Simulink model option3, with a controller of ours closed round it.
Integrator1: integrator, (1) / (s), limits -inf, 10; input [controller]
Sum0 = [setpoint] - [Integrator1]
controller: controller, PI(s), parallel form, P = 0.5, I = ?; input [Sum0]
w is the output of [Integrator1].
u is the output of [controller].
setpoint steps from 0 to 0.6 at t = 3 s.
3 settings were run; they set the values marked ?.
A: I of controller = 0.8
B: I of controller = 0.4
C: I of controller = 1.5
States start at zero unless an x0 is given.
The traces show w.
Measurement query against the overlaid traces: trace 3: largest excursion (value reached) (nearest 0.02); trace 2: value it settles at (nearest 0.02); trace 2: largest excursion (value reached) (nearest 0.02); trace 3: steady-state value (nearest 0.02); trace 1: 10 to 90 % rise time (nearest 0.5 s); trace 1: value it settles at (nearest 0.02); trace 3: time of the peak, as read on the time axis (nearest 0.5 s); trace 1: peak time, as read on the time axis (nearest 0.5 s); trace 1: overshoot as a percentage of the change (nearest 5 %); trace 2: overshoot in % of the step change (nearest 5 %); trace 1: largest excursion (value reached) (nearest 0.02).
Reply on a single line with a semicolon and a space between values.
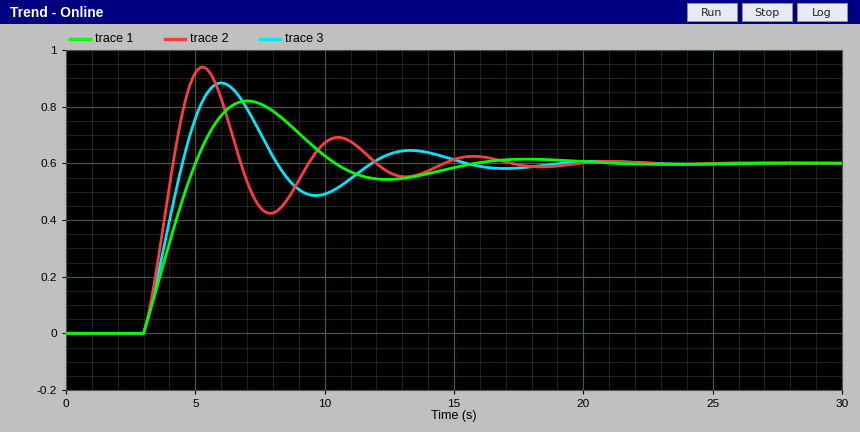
0.88; 0.60; 0.94; 0.60; 1.5 s; 0.60; 6.0 s; 7.0 s; 35 %; 55 %; 0.82
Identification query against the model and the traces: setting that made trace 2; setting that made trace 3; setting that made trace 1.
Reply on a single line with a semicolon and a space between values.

C; A; B
